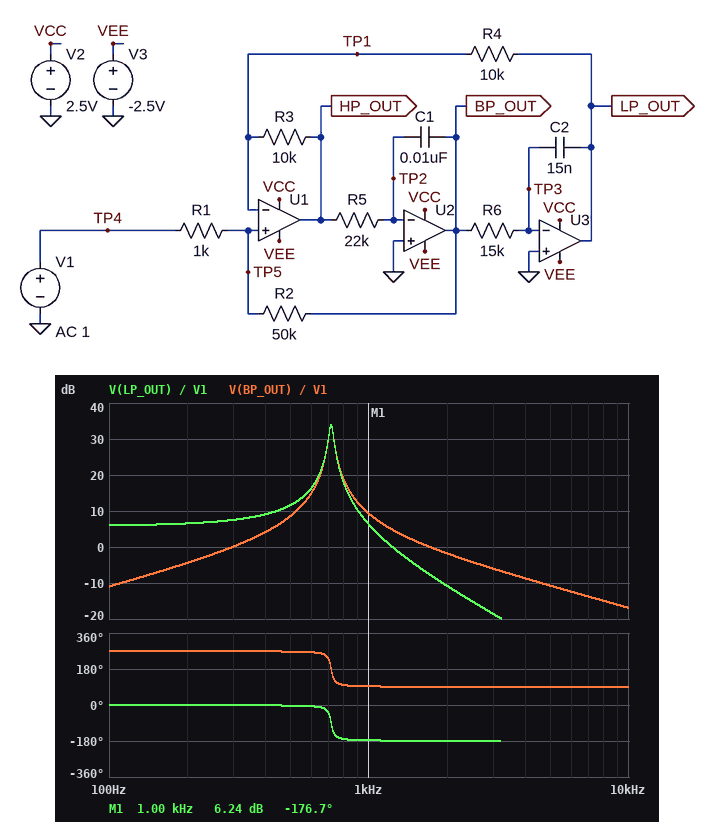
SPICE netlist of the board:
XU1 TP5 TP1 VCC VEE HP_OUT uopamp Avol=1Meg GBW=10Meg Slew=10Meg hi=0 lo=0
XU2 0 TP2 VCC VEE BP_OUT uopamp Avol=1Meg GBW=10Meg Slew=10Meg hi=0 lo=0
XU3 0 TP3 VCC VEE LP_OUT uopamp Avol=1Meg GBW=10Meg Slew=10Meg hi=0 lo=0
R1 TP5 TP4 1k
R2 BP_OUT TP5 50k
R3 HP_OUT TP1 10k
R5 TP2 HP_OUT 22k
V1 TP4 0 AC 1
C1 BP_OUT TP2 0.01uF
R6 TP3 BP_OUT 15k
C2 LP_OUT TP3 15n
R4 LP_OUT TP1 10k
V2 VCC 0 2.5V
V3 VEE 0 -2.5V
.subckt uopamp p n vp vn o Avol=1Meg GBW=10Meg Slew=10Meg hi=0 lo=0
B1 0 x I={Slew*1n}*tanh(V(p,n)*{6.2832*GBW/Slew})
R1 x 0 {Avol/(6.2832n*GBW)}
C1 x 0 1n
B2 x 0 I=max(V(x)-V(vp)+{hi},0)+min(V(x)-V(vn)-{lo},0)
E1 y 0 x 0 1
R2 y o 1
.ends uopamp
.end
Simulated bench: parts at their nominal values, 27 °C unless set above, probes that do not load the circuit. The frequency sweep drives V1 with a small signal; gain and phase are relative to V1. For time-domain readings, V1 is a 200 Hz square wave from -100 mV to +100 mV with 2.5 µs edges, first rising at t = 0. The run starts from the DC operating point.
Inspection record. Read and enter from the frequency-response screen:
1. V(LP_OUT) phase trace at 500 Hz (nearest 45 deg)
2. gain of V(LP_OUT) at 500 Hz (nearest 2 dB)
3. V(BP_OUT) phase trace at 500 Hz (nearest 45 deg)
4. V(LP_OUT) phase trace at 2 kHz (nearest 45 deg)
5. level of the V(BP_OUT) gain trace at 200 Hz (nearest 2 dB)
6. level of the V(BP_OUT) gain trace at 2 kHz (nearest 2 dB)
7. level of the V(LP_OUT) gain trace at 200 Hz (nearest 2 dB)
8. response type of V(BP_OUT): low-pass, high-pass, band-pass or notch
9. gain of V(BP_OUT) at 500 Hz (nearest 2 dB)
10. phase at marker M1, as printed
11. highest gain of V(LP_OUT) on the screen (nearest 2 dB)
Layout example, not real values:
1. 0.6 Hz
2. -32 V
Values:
1. 0 deg
2. 12 dB
3. 270 deg
4. -180 deg
5. -4 dB
6. -2 dB
7. 6 dB
8. band-pass
9. 8 dB
10. -176.7 deg
11. 34 dB
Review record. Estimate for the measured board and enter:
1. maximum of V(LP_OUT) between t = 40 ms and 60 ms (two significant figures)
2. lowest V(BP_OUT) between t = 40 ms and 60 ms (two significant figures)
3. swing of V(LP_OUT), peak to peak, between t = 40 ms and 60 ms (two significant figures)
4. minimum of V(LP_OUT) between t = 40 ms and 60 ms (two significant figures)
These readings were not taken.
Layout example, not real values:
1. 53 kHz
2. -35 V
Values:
1. 460 mV
2. -280 mV
3. 920 mV
4. -460 mV
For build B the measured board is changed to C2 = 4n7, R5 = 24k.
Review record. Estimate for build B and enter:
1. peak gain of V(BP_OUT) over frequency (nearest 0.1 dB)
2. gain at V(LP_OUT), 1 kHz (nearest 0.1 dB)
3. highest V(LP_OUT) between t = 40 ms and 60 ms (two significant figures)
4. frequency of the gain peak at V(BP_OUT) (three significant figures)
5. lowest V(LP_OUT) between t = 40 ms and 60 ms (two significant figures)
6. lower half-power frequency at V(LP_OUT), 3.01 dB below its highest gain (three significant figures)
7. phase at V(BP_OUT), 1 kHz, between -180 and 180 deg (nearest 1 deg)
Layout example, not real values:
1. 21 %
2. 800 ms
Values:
1. 34.2 dB
2. 15.4 dB
3. 410 mV
4. 1.22 kHz
5. -410 mV
6. 1.21 kHz
7. -93 deg
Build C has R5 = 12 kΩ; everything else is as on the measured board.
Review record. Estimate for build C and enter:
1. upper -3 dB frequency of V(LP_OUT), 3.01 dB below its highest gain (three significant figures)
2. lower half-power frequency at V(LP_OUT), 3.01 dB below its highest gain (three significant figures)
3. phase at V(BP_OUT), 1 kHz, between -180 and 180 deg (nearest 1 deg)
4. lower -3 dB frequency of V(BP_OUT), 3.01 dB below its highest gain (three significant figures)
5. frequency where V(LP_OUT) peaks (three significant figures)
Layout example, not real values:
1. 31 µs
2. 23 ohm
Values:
1. 993 Hz
2. 942 Hz
3. 130 deg
4. 943 Hz
5. 968 Hz
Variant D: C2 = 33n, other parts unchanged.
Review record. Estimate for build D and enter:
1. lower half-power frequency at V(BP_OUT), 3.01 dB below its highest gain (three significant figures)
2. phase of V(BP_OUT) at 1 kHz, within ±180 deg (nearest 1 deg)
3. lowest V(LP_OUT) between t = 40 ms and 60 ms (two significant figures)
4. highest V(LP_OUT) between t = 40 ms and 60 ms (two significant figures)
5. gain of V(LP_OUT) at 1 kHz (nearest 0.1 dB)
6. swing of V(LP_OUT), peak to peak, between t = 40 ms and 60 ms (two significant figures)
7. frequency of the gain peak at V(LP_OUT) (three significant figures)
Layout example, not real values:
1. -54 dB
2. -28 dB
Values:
1. 468 Hz
2. 92 deg
3. -440 mV
4. 440 mV
5. -4.5 dB
6. 880 mV
7. 482 Hz
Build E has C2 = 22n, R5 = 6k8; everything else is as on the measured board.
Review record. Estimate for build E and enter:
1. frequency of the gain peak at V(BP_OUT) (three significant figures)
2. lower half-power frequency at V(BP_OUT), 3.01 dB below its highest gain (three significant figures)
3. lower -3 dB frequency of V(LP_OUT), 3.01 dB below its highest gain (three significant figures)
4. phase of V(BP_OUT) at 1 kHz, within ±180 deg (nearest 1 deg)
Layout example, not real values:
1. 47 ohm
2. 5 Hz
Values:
1. 1.06 kHz
2. 1.02 kHz
3. 1.01 kHz
4. -125 deg
